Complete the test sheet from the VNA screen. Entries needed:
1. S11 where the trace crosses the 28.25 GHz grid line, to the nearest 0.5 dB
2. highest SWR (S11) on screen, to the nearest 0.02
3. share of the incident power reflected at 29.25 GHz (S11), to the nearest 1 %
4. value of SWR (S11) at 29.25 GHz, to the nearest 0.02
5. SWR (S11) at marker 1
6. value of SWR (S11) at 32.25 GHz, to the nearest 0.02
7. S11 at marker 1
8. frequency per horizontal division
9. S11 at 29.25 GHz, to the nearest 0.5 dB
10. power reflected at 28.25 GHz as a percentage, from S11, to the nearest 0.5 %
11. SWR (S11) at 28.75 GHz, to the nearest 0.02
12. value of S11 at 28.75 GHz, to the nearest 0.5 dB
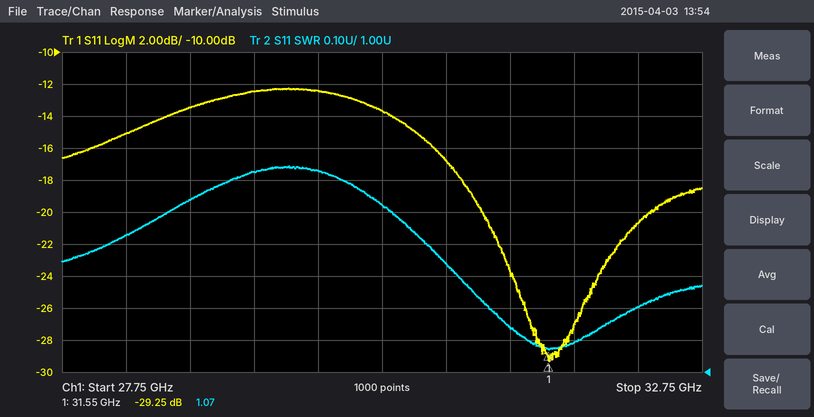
-15.0 dB
1.64
6 %
1.62
1.07
1.20
-29.25 dB
500 MHz
-12.5 dB
3.0 %
1.54
-13.5 dB
